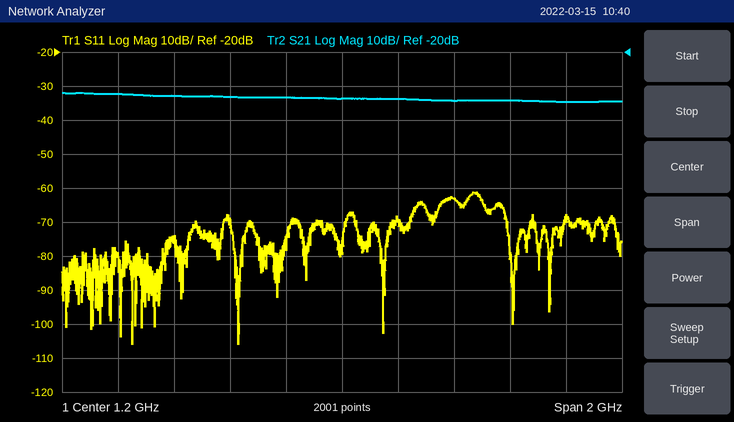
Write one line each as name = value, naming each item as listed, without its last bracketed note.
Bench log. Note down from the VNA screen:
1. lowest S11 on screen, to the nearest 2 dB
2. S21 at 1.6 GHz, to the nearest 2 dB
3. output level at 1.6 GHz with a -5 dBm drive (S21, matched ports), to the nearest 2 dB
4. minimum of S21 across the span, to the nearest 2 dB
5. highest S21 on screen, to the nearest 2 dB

lowest S11 on screen, to the nearest 2 dB = -106 dB
S21 at 1.6 GHz, to the nearest 2 dB = -34 dB
output level at 1.6 GHz with a -5 dBm drive (S21, matched ports), to the nearest 2 dB = -40 dBm
minimum of S21 across the span, to the nearest 2 dB = -34 dB
highest S21 on screen, to the nearest 2 dB = -32 dB
